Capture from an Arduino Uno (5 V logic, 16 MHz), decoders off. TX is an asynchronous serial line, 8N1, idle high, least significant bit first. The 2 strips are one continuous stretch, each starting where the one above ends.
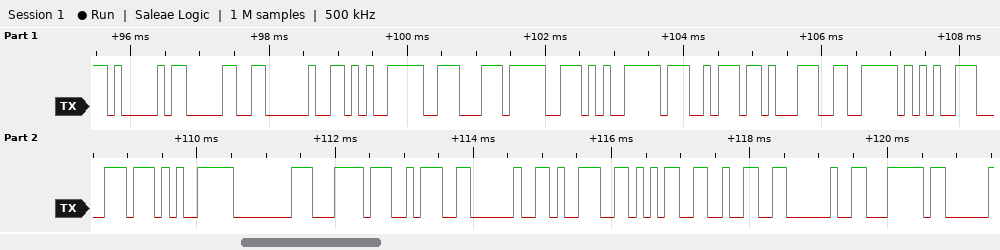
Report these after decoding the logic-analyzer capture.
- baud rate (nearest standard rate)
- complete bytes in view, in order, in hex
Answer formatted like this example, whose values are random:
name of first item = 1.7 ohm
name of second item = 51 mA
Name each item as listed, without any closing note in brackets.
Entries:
baud rate = 9600 baud
complete bytes in view, in order, in hex = 0x41 0x30 0x20 0xE5 0x8E 0x9F 0xE5 0xA7 0x8B 0xE6 0x95 0xB8 0xE5 0x80 0xBC 0x3A 0x20 0x39 0x35 0x32 0x20 0x7C
